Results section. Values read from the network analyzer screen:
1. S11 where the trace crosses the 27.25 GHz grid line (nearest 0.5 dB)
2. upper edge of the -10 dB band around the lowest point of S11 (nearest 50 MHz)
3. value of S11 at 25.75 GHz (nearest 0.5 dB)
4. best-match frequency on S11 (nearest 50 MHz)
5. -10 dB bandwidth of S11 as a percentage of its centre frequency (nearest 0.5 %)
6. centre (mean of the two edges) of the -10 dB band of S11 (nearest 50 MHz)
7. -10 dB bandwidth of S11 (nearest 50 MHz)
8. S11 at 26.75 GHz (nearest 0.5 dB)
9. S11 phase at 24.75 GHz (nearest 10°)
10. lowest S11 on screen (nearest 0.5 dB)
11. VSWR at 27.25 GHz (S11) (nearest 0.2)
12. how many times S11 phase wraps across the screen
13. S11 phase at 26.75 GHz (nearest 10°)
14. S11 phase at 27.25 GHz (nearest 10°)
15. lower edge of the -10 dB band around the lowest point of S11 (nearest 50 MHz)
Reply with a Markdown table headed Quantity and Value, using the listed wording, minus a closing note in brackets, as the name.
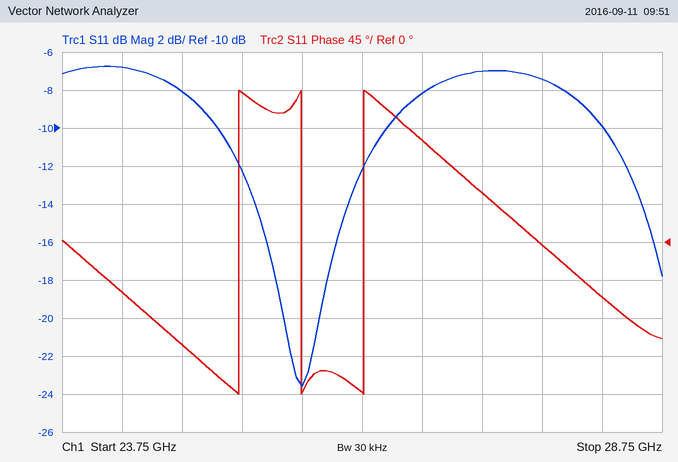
| Quantity | Value |
|---|---|
| S11 where the trace crosses the 27.25 GHz grid line | -7.0 dB |
| upper edge of the -10 dB band around the lowest point of S11 | 26.45 GHz |
| value of S11 at 25.75 GHz | -23.5 dB |
| best-match frequency on S11 | 25.75 GHz |
| -10 dB bandwidth of S11 as a percentage of its centre frequency | 5.5 % |
| centre (mean of the two edges) of the -10 dB band of S11 | 25.75 GHz |
| -10 dB bandwidth of S11 | 1.40 GHz |
| S11 at 26.75 GHz | -8.0 dB |
| S11 phase at 24.75 GHz | -120° |
| lowest S11 on screen | -23.5 dB |
| VSWR at 27.25 GHz (S11) | 2.6 |
| how many times S11 phase wraps across the screen | 3 |
| S11 phase at 26.75 GHz | 120° |
| S11 phase at 27.25 GHz | 60° |
| lower edge of the -10 dB band around the lowest point of S11 | 25.05 GHz |
